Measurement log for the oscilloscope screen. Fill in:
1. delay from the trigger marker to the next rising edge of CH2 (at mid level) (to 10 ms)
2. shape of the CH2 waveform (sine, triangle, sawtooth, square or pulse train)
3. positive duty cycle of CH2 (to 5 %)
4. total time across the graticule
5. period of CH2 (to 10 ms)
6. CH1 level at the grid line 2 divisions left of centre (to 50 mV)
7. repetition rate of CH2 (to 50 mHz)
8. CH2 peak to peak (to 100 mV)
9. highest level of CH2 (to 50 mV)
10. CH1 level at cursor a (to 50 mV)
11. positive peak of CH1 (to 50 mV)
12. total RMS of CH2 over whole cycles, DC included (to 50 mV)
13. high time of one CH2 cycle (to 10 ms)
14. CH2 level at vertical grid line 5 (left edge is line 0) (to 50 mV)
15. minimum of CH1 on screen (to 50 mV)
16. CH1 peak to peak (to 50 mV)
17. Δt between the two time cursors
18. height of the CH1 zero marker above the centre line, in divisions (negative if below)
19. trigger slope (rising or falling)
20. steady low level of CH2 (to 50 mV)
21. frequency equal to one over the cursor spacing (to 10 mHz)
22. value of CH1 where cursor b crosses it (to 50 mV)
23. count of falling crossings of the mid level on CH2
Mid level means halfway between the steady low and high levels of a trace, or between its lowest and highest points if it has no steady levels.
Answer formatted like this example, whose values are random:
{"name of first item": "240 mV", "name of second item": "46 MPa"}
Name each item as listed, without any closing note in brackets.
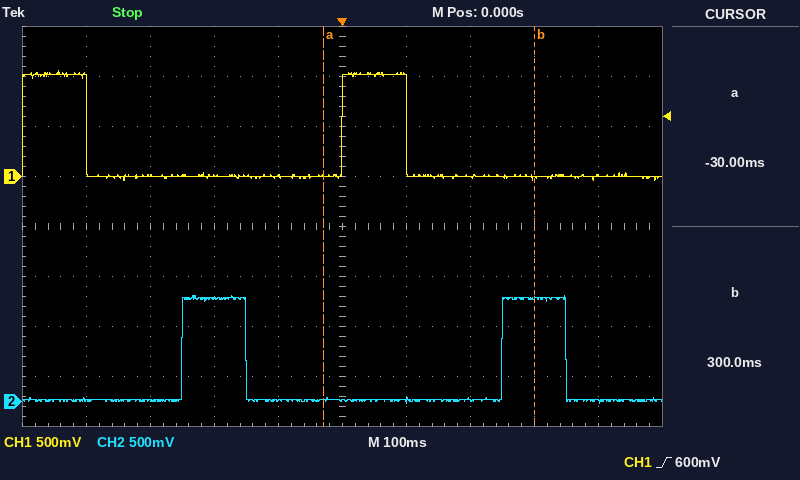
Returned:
{"delay from the trigger marker to the next rising edge of CH2 (at mid level)": "250 ms", "shape of the CH2 waveform": "pulse train", "positive duty cycle of CH2": "20 %", "total time across the graticule": "1 s", "period of CH2": "500 ms", "CH1 level at the grid line 2 divisions left of centre": "0 mV", "repetition rate of CH2": "2.00 Hz", "CH2 peak to peak": "1.10 V", "highest level of CH2": "1.05 V", "CH1 level at cursor a": "0 mV", "positive peak of CH1": "1.05 V", "total RMS of CH2 over whole cycles, DC included": "450 mV", "high time of one CH2 cycle": "100 ms", "CH2 level at vertical grid line 5 (left edge is line 0)": "0 mV", "minimum of CH1 on screen": "-50 mV", "CH1 peak to peak": "1.10 V", "Δt between the two time cursors": "330 ms", "height of the CH1 zero marker above the centre line, in divisions": "+1.0 div", "trigger slope": "rising", "steady low level of CH2": "0 mV", "frequency equal to one over the cursor spacing": "3.03 Hz", "value of CH1 where cursor b crosses it": "0 mV", "count of falling crossings of the mid level on CH2": "2"}
